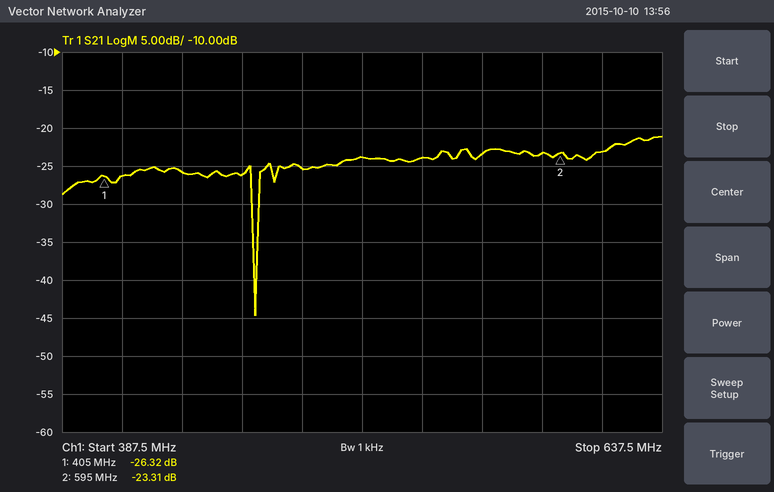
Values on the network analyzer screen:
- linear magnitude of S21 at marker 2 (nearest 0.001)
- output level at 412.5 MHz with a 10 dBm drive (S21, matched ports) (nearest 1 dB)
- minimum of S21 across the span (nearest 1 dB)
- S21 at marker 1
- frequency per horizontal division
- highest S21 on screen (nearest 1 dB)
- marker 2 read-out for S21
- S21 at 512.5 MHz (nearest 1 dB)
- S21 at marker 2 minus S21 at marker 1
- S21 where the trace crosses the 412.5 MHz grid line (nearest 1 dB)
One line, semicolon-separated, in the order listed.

0.068; -16 dBm; -45 dB; -26.32 dB; 25 MHz; -21 dB; -23.31 dB; -24 dB; 3.01 dB; -26 dB
